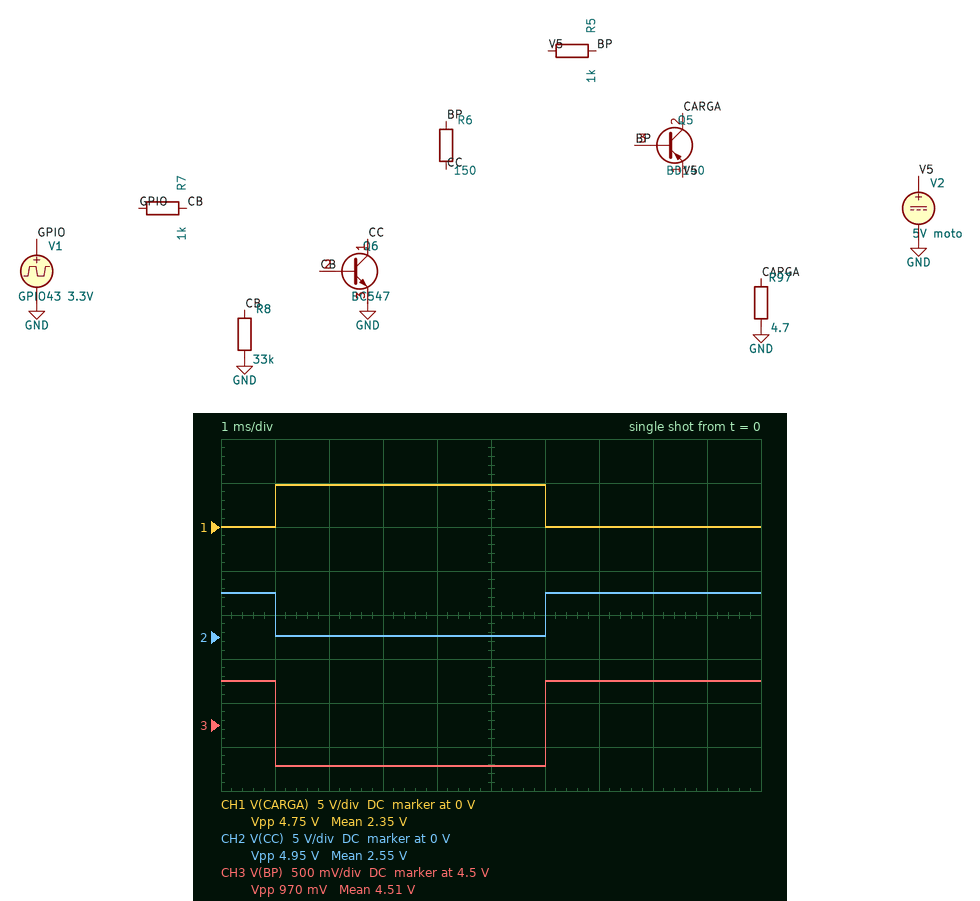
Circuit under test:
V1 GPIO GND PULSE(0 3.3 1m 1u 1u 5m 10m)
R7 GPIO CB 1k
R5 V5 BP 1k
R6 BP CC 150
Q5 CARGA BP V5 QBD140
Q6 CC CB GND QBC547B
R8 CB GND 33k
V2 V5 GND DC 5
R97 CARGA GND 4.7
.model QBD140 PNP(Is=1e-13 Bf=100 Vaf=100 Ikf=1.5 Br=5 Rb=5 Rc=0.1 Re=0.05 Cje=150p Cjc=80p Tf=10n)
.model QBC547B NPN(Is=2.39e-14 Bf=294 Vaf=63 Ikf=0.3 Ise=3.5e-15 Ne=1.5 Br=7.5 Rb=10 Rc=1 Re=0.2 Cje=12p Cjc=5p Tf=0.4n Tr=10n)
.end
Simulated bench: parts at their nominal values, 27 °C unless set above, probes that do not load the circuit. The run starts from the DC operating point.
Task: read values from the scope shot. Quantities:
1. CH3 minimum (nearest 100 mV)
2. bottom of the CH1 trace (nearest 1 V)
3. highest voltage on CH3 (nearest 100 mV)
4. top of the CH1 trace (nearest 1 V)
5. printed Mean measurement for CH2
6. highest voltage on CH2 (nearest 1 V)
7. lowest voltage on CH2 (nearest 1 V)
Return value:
4.0 V
0 V
5.0 V
5 V
2.55 V
5 V
0 V
